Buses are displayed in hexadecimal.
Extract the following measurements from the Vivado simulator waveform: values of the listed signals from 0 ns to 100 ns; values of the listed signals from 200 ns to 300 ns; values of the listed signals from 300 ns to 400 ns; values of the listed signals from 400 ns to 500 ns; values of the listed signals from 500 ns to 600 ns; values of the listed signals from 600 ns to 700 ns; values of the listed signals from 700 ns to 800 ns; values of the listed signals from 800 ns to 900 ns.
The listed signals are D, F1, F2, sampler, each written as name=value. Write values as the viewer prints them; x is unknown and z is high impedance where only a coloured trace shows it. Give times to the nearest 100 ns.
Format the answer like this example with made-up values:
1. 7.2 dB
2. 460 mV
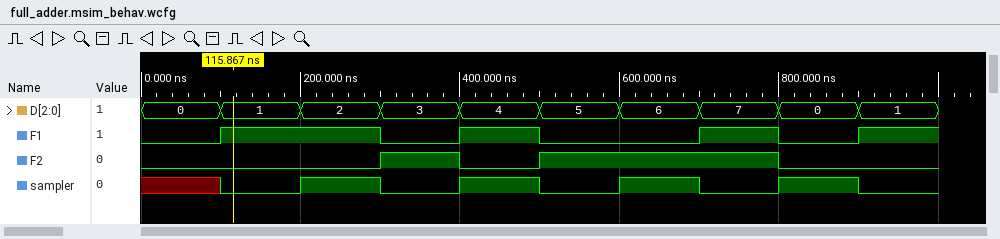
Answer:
1. D=0, F1=0, F2=0, sampler=x
2. D=2, F1=1, F2=0, sampler=1
3. D=3, F1=0, F2=1, sampler=0
4. D=4, F1=1, F2=0, sampler=1
5. D=5, F1=0, F2=1, sampler=0
6. D=6, F1=0, F2=1, sampler=1
7. D=7, F1=1, F2=1, sampler=0
8. D=0, F1=0, F2=0, sampler=1
